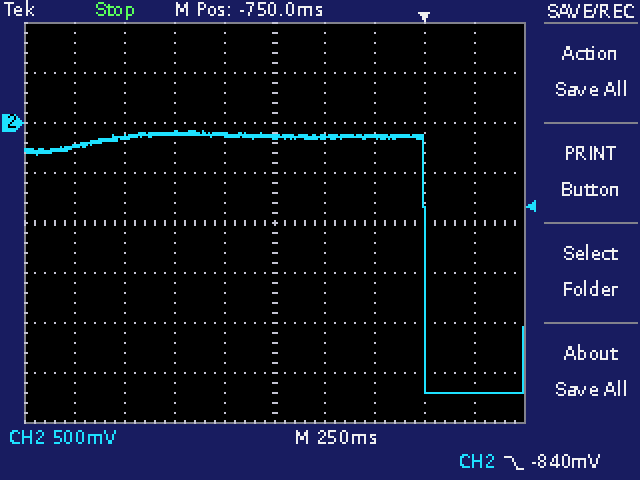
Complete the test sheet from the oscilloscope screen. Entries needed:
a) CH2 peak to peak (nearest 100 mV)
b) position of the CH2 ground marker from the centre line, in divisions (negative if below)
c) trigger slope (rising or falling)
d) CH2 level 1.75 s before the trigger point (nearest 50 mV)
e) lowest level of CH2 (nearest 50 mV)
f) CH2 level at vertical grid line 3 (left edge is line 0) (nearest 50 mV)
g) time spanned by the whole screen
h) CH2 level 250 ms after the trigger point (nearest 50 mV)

2.60 V
+2.0 div
falling
-250 mV
-2.70 V
-100 mV
2.5 s
-2.70 V
